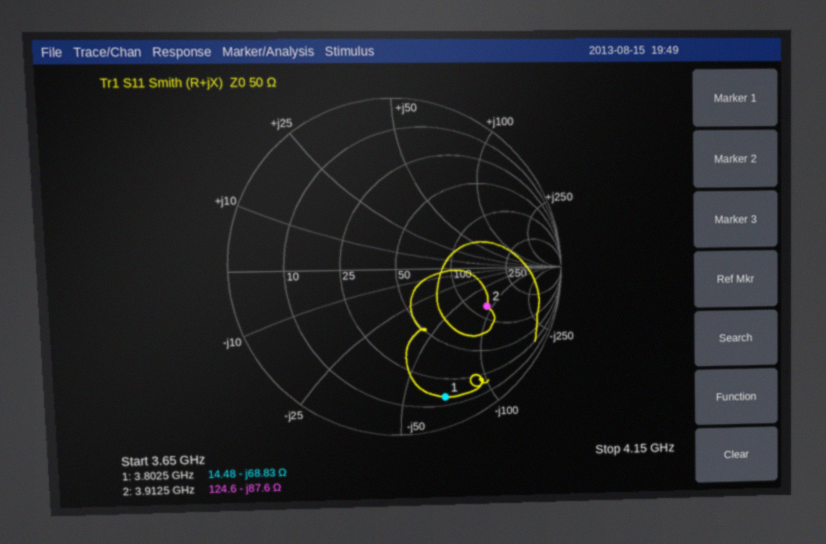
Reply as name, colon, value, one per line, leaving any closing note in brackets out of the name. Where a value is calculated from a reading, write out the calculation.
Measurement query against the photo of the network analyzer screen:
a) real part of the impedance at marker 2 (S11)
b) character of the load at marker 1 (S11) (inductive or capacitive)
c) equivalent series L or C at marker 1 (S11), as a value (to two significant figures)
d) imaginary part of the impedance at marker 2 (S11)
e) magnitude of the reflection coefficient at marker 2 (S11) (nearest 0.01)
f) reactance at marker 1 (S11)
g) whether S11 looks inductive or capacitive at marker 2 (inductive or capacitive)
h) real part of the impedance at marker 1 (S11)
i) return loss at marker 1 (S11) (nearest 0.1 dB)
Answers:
real part of the impedance at marker 2: 124.6 Ω
character of the load at marker 1 (S11): capacitive
equivalent series L or C at marker 1 (S11), as a value: C = 1/(2π × 3.8025 GHz × 68.83 Ω) ≈ 608 fF, so 610 fF to two significant figures
imaginary part of the impedance at marker 2: -87.6 Ω
magnitude of the reflection coefficient at marker 2 (S11): 0.59
reactance at marker 1: -68.83 Ω
whether S11 looks inductive or capacitive at marker 2: capacitive
real part of the impedance at marker 1: 14.48 Ω
return loss at marker 1 (S11): 1.7 dB
